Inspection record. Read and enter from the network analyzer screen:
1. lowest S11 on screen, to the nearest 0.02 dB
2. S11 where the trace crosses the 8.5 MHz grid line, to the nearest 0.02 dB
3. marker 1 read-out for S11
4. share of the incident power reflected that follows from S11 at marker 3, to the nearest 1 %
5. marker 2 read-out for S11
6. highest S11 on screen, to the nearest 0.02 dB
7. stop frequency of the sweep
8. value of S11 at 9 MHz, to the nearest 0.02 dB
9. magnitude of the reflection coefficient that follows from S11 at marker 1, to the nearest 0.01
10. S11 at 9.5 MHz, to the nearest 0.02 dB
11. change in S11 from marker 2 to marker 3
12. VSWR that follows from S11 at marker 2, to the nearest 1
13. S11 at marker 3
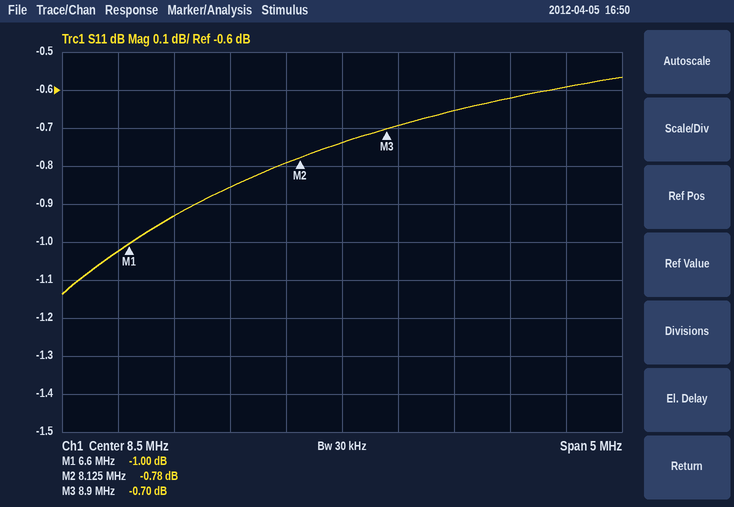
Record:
-1.14 dB
-0.74 dB
-1.00 dB
85 %
-0.78 dB
-0.56 dB
11 MHz
-0.70 dB
0.89
-0.66 dB
0.08 dB
22
-0.70 dB
